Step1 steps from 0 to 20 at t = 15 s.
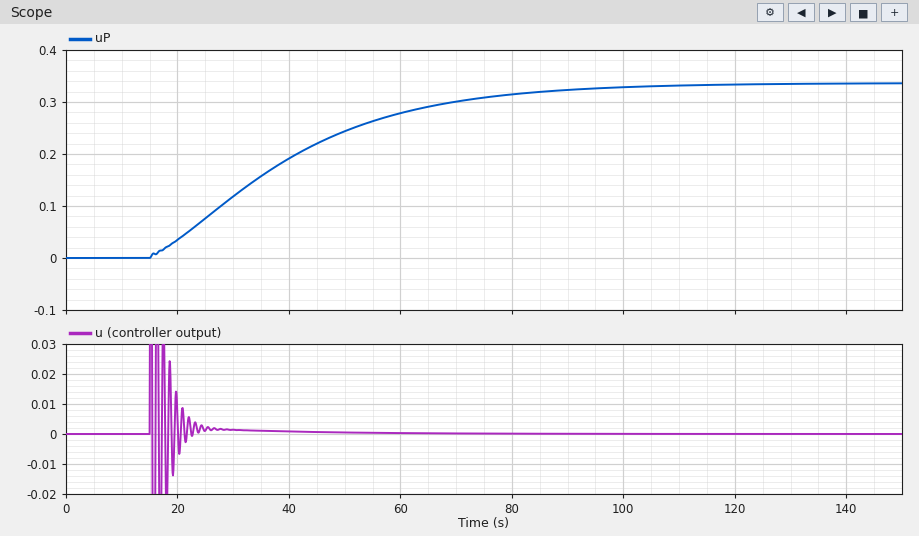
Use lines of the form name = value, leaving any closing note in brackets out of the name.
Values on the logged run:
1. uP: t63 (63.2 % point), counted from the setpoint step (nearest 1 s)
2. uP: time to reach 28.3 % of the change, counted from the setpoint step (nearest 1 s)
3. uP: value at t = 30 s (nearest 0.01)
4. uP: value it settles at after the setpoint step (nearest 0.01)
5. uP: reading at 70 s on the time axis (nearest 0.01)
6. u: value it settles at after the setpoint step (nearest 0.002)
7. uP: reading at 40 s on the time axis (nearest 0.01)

uP: t63 (63.2 % point), counted from the setpoint step = 29 s
uP: time to reach 28.3 % of the change, counted from the setpoint step = 12 s
uP: value at t = 30 s = 0.12
uP: value it settles at after the setpoint step = 0.34
uP: reading at 70 s on the time axis = 0.30
u: value it settles at after the setpoint step = 0.000
uP: reading at 40 s on the time axis = 0.19
